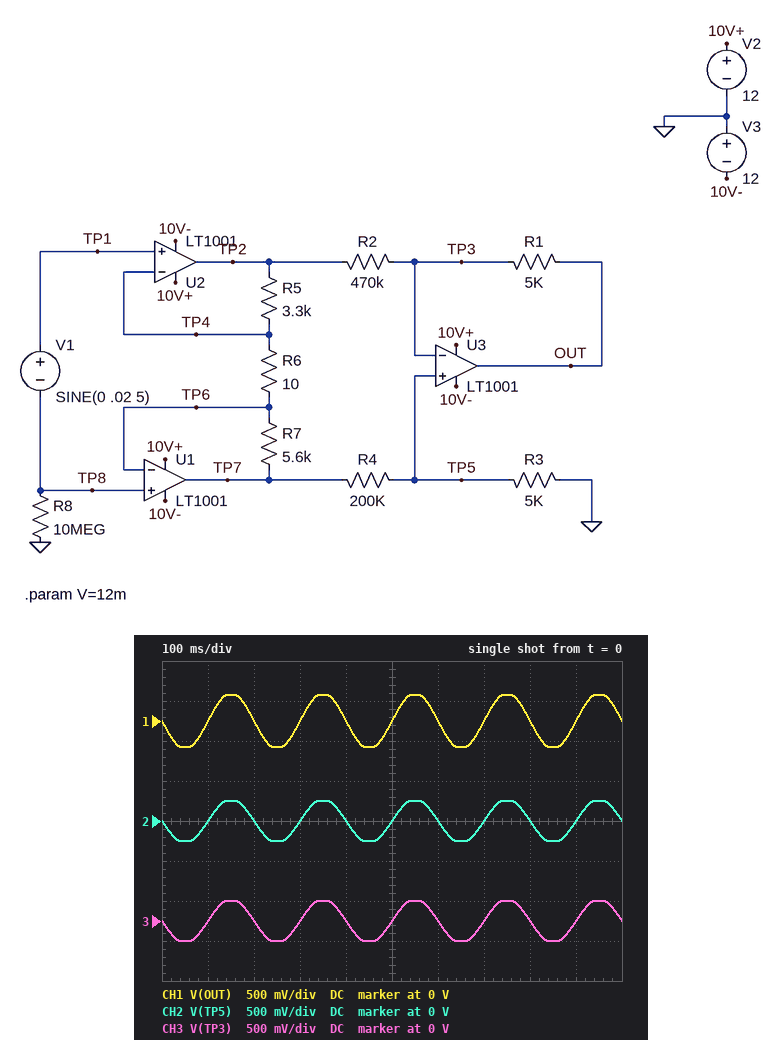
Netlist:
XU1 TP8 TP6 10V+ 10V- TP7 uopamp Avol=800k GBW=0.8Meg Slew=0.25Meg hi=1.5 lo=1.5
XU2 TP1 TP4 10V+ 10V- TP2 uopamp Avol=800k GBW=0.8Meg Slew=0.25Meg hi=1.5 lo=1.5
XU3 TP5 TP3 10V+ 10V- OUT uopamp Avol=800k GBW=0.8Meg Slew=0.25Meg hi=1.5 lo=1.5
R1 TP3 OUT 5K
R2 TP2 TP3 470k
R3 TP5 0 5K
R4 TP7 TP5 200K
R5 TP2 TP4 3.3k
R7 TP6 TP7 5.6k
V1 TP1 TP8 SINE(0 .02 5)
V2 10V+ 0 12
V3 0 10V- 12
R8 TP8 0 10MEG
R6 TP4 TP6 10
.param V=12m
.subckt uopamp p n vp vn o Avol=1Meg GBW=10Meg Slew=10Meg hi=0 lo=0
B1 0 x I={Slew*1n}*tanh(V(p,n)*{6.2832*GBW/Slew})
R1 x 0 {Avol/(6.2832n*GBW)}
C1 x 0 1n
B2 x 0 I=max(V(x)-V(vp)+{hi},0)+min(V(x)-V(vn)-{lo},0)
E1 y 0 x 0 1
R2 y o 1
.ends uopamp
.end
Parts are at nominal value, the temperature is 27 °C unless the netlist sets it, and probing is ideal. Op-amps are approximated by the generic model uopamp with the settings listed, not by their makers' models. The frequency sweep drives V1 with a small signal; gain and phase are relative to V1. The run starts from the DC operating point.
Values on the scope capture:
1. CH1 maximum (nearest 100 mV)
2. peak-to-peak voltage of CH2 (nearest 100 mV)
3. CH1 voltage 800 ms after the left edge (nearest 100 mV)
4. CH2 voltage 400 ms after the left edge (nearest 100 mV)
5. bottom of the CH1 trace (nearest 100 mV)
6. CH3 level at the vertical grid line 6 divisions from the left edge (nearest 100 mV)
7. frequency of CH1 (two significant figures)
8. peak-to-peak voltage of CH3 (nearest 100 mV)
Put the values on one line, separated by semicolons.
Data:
300 mV; 500 mV; 0 V; 0 V; -300 mV; 0 V; 5.0 Hz; 500 mV
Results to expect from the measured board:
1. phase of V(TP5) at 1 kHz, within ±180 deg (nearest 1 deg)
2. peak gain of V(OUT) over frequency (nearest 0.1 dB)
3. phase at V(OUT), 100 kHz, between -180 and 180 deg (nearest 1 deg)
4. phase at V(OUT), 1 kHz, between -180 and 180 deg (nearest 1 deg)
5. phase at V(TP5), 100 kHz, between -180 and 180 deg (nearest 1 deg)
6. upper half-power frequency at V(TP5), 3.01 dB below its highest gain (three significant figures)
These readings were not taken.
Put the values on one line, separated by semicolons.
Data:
132 deg; 24.8 dB; 80 deg; 132 deg; 83 deg; 899 Hz
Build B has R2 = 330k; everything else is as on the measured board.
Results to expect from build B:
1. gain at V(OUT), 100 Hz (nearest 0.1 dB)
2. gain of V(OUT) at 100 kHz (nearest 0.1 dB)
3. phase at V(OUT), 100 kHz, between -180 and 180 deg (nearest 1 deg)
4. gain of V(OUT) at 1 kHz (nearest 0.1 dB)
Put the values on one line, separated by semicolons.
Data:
25.5 dB; -15.5 dB; 81 deg; 22.0 dB
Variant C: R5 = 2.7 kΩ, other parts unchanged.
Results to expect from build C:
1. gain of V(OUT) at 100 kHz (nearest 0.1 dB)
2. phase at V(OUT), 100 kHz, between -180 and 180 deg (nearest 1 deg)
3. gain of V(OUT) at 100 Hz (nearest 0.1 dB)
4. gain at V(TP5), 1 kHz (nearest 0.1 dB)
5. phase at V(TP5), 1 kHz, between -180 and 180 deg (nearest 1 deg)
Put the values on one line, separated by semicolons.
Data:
-16.0 dB; 80 deg; 24.4 dB; 19.5 dB; 134 deg
